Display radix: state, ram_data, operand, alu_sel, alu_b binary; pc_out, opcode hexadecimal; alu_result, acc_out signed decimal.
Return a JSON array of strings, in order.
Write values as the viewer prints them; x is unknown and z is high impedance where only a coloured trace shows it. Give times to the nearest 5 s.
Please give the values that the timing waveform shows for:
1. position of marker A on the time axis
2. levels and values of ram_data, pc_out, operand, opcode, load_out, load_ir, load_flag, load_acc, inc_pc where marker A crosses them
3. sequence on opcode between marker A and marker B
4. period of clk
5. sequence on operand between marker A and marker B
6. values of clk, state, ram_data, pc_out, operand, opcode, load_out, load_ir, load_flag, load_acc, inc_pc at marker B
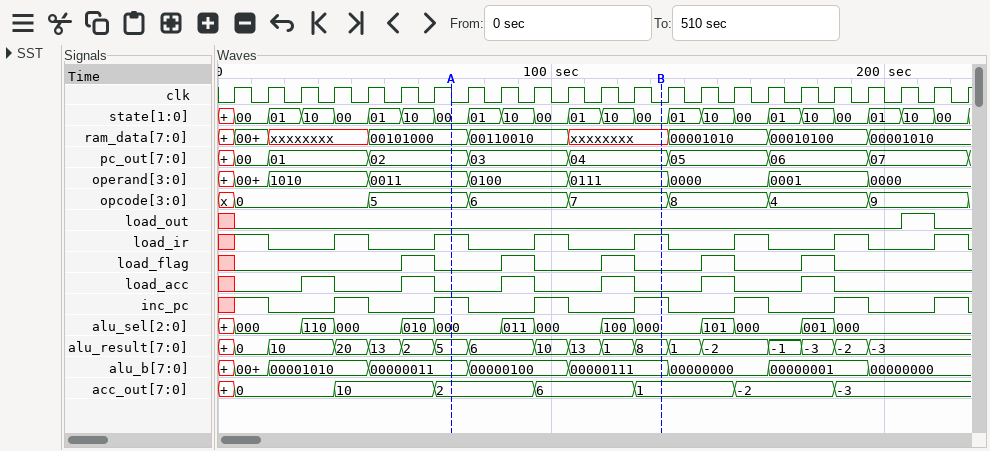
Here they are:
["70 s", "ram_data=00101000, pc_out=02, operand=0011, opcode=5, load_out=0, load_ir=1, load_flag=0, load_acc=0, inc_pc=1", "5, 6, 7", "10 s", "0011, 0100, 0111", "clk=0, state=00, ram_data=xxxxxxxx, pc_out=04, operand=0111, opcode=7, load_out=0, load_ir=1, load_flag=0, load_acc=0, inc_pc=1"]
